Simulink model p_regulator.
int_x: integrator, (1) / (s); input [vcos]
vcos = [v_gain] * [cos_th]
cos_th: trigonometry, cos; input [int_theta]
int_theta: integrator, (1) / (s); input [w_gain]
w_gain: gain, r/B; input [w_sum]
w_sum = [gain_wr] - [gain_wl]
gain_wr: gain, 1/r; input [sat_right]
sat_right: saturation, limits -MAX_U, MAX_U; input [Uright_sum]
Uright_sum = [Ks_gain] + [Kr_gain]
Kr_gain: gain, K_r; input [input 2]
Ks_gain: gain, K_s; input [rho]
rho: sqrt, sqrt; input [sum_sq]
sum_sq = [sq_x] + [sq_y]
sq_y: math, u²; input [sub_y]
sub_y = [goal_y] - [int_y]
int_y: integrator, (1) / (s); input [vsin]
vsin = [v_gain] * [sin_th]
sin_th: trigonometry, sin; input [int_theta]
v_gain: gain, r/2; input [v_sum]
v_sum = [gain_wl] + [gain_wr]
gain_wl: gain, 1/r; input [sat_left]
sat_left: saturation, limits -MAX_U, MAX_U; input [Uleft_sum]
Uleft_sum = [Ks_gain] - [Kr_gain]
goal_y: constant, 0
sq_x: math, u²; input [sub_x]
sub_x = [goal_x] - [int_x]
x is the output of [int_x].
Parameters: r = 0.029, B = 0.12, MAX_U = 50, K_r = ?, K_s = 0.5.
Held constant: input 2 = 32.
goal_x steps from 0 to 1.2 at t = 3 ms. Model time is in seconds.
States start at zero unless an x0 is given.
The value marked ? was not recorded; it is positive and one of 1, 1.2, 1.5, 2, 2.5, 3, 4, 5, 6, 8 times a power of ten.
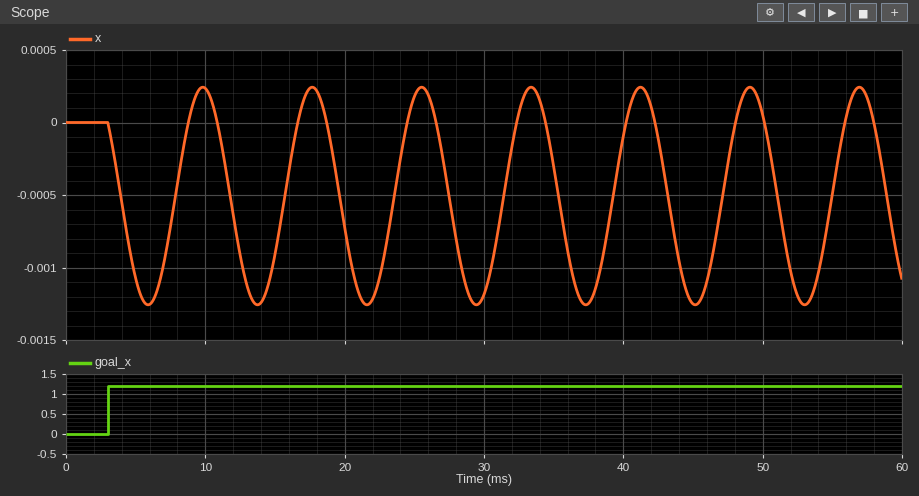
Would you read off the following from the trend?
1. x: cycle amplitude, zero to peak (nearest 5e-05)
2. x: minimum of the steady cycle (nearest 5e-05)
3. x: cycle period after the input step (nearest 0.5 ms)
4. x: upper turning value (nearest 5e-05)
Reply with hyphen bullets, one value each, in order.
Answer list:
- 0.00075
- -0.00125
- 8.0 ms
- 0.00025
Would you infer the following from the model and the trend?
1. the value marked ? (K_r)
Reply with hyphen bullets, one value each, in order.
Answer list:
- 1.5
